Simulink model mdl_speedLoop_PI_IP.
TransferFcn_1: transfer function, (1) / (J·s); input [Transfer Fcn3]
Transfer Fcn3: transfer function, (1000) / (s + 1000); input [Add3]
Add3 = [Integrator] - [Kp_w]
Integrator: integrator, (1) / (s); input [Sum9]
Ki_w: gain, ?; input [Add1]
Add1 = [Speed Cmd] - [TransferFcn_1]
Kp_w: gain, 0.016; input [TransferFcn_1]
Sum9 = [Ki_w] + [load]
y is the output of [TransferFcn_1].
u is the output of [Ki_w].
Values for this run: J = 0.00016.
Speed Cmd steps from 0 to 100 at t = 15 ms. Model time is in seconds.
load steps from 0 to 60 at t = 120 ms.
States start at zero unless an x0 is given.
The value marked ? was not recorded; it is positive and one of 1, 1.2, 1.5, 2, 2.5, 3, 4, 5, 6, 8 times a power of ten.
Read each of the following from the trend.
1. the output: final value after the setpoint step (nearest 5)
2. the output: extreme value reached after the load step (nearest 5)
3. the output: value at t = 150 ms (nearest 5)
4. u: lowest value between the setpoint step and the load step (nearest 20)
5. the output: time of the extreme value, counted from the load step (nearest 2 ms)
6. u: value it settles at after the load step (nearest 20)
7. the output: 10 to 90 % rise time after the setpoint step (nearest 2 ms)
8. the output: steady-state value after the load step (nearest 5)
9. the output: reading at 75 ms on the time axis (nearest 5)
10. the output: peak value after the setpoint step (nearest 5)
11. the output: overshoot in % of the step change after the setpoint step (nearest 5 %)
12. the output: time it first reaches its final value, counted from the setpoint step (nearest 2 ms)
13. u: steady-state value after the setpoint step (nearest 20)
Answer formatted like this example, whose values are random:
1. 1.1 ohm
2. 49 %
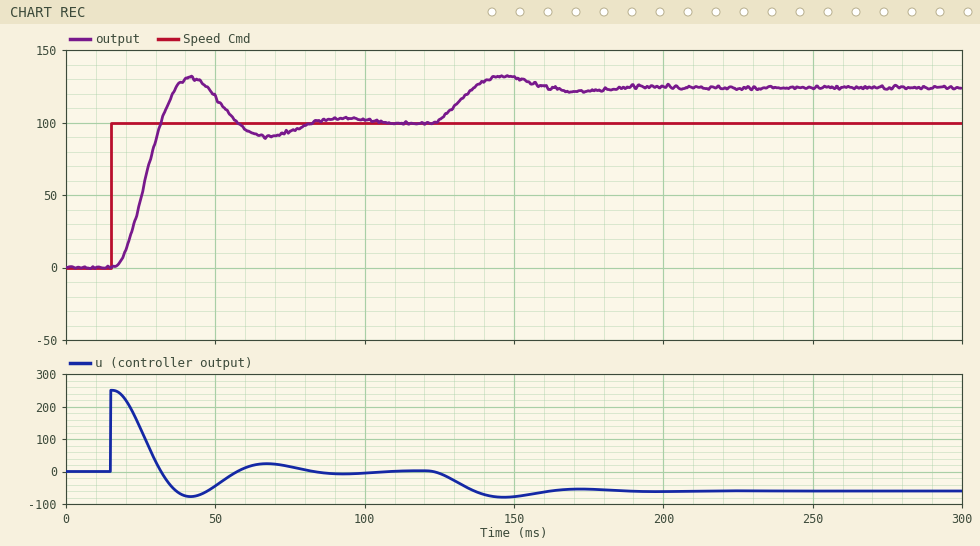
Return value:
1. 100
2. 130
3. 130
4. -80
5. 26 ms
6. -60
7. 10 ms
8. 125
9. 95
10. 130
11. 30 %
12. 16 ms
13. 0
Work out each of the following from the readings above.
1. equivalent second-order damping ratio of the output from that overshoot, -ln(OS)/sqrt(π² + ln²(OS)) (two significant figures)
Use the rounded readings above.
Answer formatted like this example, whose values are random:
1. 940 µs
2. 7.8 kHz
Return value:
1. 0.36
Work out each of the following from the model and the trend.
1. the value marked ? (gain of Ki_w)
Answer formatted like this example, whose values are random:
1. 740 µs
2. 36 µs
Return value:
1. 2.5
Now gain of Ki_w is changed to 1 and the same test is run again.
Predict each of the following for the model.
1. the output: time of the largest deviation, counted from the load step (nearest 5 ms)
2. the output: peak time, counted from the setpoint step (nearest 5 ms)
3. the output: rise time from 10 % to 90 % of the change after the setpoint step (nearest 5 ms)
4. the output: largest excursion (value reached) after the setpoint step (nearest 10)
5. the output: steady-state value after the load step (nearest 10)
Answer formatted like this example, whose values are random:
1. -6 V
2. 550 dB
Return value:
1. 50 ms
2. 50 ms
3. 25 ms
4. 110
5. 160
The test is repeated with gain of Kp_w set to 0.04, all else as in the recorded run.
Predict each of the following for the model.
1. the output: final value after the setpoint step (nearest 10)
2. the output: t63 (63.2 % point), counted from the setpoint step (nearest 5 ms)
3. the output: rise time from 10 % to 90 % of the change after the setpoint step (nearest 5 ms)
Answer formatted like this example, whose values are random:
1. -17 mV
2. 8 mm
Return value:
1. 100
2. 15 ms
3. 25 ms
